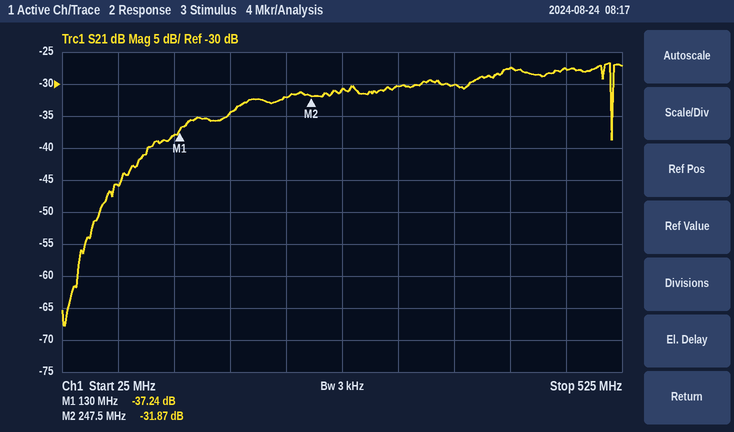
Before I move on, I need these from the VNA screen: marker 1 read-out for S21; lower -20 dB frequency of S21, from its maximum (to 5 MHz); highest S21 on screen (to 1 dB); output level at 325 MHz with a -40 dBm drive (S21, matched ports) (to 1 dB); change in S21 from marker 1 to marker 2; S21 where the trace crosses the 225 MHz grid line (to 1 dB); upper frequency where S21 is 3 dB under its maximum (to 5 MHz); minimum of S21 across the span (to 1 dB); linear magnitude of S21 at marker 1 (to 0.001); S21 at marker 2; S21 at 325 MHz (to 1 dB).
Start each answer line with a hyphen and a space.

- -37.24 dB
- 70 MHz
- -27 dB
- -70 dBm
- 5.37 dB
- -32 dB
- 515 MHz
- -68 dB
- 0.014
- -31.87 dB
- -30 dB
